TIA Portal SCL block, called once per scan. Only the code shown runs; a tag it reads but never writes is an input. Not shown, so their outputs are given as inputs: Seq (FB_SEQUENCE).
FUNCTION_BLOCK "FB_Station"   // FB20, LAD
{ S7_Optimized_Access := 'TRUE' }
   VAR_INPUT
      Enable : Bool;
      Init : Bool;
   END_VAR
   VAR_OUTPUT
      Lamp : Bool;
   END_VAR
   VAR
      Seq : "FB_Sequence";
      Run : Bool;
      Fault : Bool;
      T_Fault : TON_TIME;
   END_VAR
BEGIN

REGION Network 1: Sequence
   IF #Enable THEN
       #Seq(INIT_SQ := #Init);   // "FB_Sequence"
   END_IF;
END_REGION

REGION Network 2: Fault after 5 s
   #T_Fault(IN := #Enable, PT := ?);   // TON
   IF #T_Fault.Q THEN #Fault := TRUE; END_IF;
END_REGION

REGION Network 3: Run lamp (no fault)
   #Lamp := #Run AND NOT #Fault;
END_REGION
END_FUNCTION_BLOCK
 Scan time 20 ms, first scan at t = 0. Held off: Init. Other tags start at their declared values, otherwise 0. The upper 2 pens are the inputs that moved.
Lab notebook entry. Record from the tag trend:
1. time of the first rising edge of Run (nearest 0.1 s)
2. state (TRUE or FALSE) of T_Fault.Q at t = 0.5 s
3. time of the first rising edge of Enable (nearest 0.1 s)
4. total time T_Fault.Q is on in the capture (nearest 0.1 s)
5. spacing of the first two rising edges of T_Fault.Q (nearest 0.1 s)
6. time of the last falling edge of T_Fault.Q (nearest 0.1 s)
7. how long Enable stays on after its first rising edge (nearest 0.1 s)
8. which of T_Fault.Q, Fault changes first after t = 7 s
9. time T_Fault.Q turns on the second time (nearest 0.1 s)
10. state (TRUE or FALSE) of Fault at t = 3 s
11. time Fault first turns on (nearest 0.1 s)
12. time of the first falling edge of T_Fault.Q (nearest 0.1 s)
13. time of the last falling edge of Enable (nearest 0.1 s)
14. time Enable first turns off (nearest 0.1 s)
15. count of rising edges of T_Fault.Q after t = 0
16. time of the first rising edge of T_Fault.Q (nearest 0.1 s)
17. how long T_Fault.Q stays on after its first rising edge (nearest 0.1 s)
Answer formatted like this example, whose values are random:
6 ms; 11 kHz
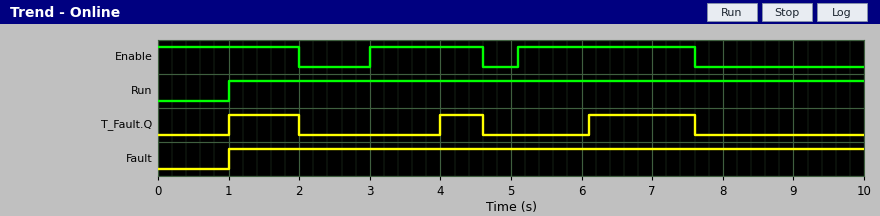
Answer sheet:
1.0 s; FALSE; 3.0 s; 3.1 s; 3.0 s; 7.6 s; 1.6 s; T_Fault.Q; 4.0 s; TRUE; 1.0 s; 2.0 s; 7.6 s; 2.0 s; 3; 1.0 s; 1.0 s
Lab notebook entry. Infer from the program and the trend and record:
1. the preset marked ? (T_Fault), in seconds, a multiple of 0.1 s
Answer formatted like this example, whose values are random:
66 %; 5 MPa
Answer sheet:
1.0 s
